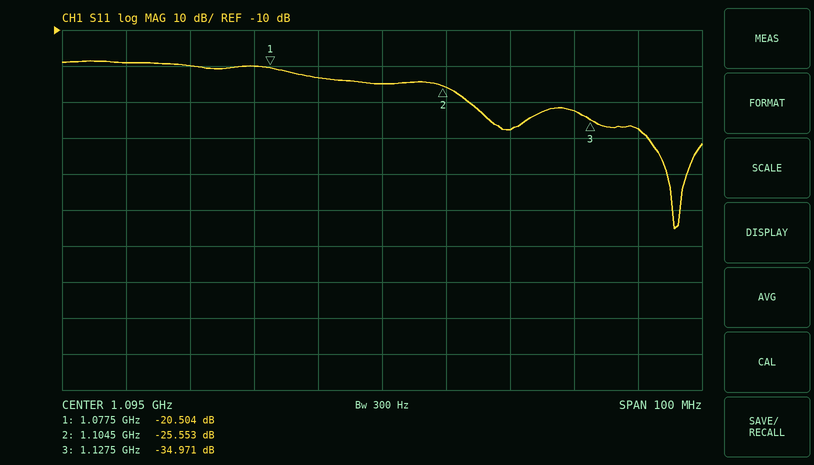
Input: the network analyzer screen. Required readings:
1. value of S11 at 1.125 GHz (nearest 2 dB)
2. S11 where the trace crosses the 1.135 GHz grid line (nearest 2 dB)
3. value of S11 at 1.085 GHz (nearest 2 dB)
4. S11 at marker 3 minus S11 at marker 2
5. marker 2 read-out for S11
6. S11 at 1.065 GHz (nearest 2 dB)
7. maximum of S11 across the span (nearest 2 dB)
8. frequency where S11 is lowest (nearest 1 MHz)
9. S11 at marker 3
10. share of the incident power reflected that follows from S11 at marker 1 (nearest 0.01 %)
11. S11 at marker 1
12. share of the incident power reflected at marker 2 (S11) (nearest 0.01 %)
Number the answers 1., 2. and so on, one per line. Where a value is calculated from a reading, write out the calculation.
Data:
1. -32 dB
2. -38 dB
3. -24 dB
4. -34.971 − (-25.553) = -9.418 dB
5. -25.553 dB
6. -20 dB
7. -18 dB
8. 1.141 GHz
9. -34.971 dB
10. 10^(-20.504/10) ≈ 0.89 %
11. -20.504 dB
12. 10^(-25.553/10) ≈ 0.28 %
